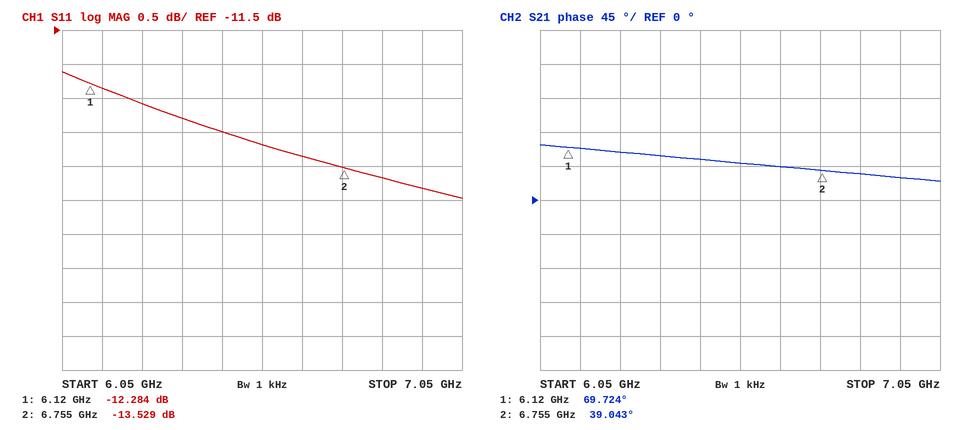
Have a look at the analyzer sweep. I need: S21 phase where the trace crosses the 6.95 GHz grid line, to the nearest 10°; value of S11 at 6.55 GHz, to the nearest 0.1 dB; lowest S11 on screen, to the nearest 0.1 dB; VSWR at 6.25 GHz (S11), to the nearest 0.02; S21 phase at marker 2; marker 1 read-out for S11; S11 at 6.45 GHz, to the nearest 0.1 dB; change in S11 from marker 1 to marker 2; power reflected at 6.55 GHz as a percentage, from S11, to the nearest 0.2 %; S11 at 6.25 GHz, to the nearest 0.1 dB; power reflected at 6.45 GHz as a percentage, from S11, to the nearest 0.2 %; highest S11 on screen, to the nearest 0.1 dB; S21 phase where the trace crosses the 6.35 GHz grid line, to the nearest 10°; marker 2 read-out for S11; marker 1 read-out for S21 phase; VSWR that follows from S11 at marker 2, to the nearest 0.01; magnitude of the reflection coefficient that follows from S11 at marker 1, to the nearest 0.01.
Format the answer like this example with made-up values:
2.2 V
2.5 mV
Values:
30°
-13.2 dB
-14.0 dB
1.62
39.043°
-12.284 dB
-13.0 dB
-1.245 dB
4.8 %
-12.6 dB
5.0 %
-12.1 dB
60°
-13.529 dB
69.724°
1.53
0.24
